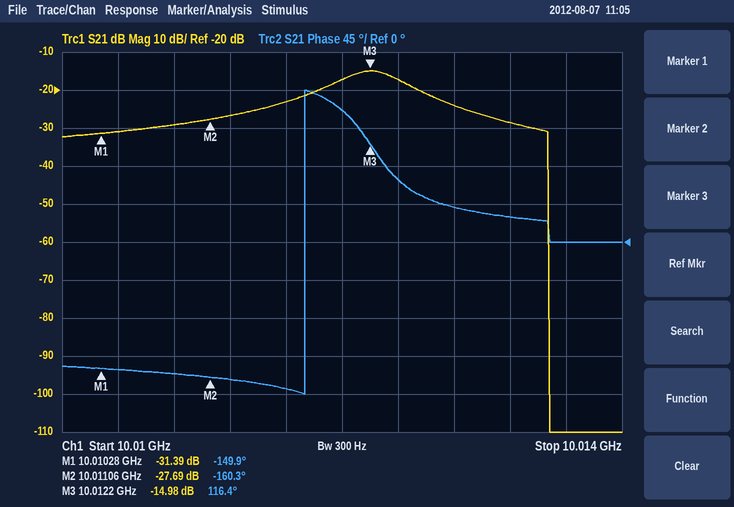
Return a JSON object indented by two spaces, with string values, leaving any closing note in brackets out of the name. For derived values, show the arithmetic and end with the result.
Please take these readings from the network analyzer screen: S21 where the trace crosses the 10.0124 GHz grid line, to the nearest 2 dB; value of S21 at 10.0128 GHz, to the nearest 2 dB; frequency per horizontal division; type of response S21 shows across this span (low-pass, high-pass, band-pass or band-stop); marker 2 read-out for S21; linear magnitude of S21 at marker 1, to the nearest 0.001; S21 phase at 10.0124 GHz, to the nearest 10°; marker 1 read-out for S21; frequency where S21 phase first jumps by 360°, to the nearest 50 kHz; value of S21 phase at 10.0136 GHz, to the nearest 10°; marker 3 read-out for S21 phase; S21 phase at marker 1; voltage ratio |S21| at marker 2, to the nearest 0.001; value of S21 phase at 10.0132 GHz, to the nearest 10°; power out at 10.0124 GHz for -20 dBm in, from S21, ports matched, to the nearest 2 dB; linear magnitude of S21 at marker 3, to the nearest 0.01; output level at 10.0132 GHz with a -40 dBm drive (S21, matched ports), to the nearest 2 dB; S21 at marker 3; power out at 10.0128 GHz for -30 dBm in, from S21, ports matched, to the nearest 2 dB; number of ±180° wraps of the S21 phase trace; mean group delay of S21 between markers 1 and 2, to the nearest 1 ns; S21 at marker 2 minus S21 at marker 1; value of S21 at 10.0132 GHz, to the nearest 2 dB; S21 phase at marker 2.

{
  "S21 where the trace crosses the 10.0124 GHz grid line, to the nearest 2 dB": "-18 dB",
  "value of S21 at 10.0128 GHz, to the nearest 2 dB": "-24 dB",
  "frequency per horizontal division": "400 kHz",
  "type of response S21 shows across this span": "band-pass",
  "marker 2 read-out for S21": "-27.69 dB",
  "linear magnitude of S21 at marker 1, to the nearest 0.001": "10^(-31.39/20) ≈ 0.027",
  "S21 phase at 10.0124 GHz, to the nearest 10°": "70°",
  "marker 1 read-out for S21": "-31.39 dB",
  "frequency where S21 phase first jumps by 360°, to the nearest 50 kHz": "10.01175 GHz",
  "value of S21 phase at 10.0136 GHz, to the nearest 10°": "0°",
  "marker 3 read-out for S21 phase": "116.4°",
  "S21 phase at marker 1": "-149.9°",
  "voltage ratio |S21| at marker 2, to the nearest 0.001": "10^(-27.69/20) ≈ 0.041",
  "value of S21 phase at 10.0132 GHz, to the nearest 10°": "30°",
  "power out at 10.0124 GHz for -20 dBm in, from S21, ports matched, to the nearest 2 dB": "-20 dBm + (-18 dB) = -38 dBm",
  "linear magnitude of S21 at marker 3, to the nearest 0.01": "10^(-14.98/20) ≈ 0.18",
  "output level at 10.0132 GHz with a -40 dBm drive (S21, matched ports), to the nearest 2 dB": "-40 dBm + (-28 dB) = -68 dBm",
  "S21 at marker 3": "-14.98 dB",
  "power out at 10.0128 GHz for -30 dBm in, from S21, ports matched, to the nearest 2 dB": "-30 dBm + (-24 dB) = -54 dBm",
  "number of ±180° wraps of the S21 phase trace": "1",
  "mean group delay of S21 between markers 1 and 2, to the nearest 1 ns": "−(-160.3° − (-149.9°))/(360° × 780 kHz) ≈ 37 ns",
  "S21 at marker 2 minus S21 at marker 1": "-27.69 − (-31.39) = 3.70 dB",
  "value of S21 at 10.0132 GHz, to the nearest 2 dB": "-28 dB",
  "S21 phase at marker 2": "-160.3°"
}
